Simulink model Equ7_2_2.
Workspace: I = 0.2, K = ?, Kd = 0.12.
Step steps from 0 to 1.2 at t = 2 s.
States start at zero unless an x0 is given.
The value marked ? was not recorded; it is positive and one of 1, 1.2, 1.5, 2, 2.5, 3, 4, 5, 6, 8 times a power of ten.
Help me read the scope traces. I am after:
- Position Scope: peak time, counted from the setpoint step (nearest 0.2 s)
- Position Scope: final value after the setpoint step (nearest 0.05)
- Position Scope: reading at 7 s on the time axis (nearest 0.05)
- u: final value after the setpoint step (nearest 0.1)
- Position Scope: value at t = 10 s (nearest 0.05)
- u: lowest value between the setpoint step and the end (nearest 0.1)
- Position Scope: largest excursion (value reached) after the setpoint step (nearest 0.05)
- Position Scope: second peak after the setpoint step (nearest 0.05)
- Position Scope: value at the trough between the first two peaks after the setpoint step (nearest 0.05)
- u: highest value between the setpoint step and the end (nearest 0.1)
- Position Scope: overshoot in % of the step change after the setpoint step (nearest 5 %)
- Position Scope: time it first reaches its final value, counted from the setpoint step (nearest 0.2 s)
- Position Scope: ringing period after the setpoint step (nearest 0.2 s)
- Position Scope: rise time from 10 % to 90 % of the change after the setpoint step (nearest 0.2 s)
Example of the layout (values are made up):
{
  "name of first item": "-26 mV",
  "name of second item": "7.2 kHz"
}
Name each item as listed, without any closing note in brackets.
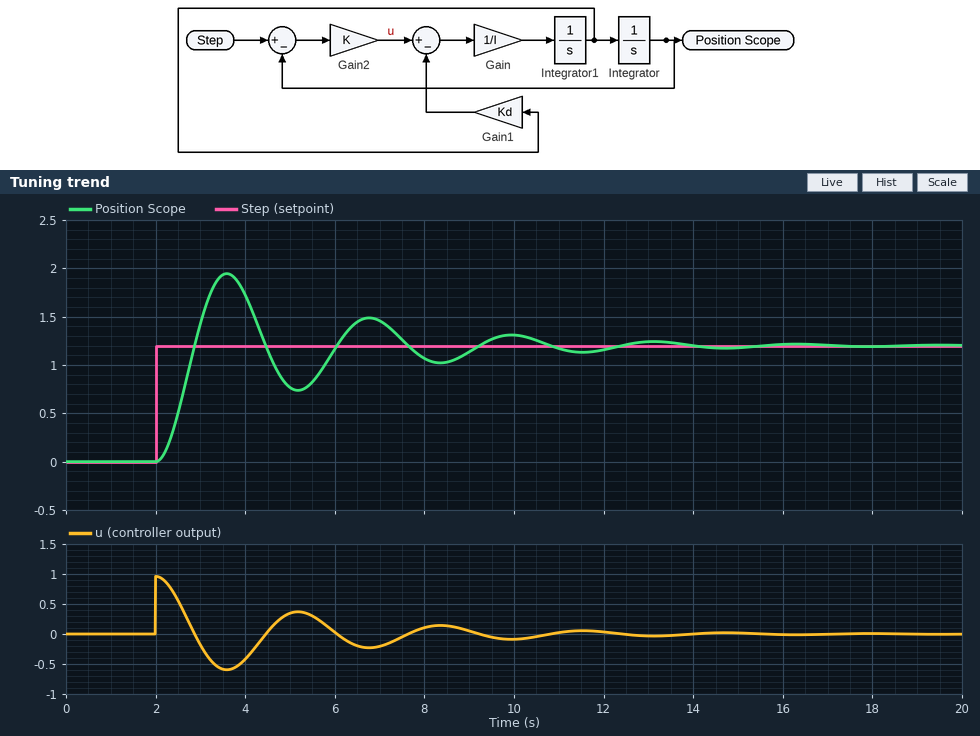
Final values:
{
  "Position Scope: peak time, counted from the setpoint step": "1.6 s",
  "Position Scope: final value after the setpoint step": "1.20",
  "Position Scope: reading at 7 s on the time axis": "1.45",
  "u: final value after the setpoint step": "0.0",
  "Position Scope: value at t = 10 s": "1.30",
  "u: lowest value between the setpoint step and the end": "-0.6",
  "Position Scope: largest excursion (value reached) after the setpoint step": "1.95",
  "Position Scope: second peak after the setpoint step": "1.50",
  "Position Scope: value at the trough between the first two peaks after the setpoint step": "0.75",
  "u: highest value between the setpoint step and the end": "1.0",
  "Position Scope: overshoot in % of the step change after the setpoint step": "60 %",
  "Position Scope: time it first reaches its final value, counted from the setpoint step": "0.8 s",
  "Position Scope: ringing period after the setpoint step": "3.2 s",
  "Position Scope: rise time from 10 % to 90 % of the change after the setpoint step": "0.6 s"
}
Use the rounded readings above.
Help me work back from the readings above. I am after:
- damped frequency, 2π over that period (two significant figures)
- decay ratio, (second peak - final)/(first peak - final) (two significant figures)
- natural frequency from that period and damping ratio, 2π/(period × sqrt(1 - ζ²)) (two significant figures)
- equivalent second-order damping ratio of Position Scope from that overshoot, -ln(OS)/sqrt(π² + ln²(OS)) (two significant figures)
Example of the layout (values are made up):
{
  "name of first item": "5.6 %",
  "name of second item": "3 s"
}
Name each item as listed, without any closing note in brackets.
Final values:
{
  "damped frequency, 2π over that period": "2.0 rad/s",
  "decay ratio, (second peak - final)/(first peak - final)": "0.40",
  "natural frequency from that period and damping ratio, 2π/(period × sqrt(1 - ζ²))": "2.0 rad/s",
  "equivalent second-order damping ratio of Position Scope from that overshoot, -ln(OS)/sqrt(π² + ln²(OS))": "0.16"
}
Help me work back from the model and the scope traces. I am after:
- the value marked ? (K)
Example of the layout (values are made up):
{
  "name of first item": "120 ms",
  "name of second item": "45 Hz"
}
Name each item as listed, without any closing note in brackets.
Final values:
{
  "the value marked ?": "0.8"
}
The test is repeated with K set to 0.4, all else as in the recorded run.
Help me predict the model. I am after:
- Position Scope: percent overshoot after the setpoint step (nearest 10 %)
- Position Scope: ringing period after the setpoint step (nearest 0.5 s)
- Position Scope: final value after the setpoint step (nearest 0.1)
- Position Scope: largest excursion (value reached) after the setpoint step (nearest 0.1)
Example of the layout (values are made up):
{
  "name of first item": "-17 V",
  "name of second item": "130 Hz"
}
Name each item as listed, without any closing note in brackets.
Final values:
{
  "Position Scope: percent overshoot after the setpoint step": "50 %",
  "Position Scope: ringing period after the setpoint step": "4.5 s",
  "Position Scope: final value after the setpoint step": "1.2",
  "Position Scope: largest excursion (value reached) after the setpoint step": "1.8"
}
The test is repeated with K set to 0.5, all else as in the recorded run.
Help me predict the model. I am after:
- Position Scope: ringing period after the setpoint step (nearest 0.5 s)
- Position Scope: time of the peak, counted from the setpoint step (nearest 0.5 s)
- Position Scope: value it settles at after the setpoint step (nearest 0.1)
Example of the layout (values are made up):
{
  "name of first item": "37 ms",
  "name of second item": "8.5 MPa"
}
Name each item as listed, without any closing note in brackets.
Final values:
{
  "Position Scope: ringing period after the setpoint step": "4.0 s",
  "Position Scope: time of the peak, counted from the setpoint step": "2.0 s",
  "Position Scope: value it settles at after the setpoint step": "1.2"
}
